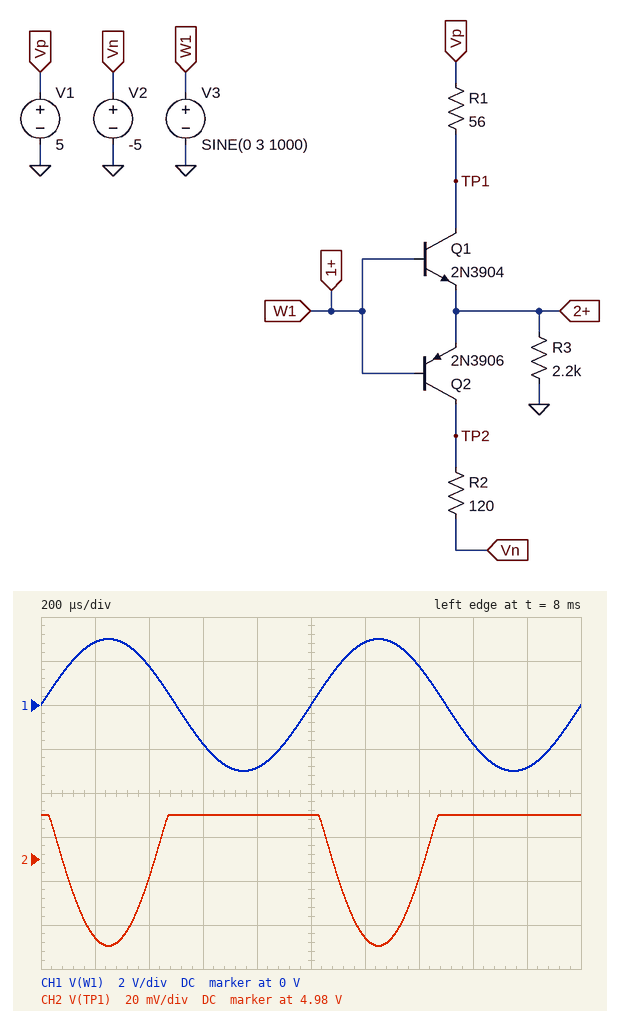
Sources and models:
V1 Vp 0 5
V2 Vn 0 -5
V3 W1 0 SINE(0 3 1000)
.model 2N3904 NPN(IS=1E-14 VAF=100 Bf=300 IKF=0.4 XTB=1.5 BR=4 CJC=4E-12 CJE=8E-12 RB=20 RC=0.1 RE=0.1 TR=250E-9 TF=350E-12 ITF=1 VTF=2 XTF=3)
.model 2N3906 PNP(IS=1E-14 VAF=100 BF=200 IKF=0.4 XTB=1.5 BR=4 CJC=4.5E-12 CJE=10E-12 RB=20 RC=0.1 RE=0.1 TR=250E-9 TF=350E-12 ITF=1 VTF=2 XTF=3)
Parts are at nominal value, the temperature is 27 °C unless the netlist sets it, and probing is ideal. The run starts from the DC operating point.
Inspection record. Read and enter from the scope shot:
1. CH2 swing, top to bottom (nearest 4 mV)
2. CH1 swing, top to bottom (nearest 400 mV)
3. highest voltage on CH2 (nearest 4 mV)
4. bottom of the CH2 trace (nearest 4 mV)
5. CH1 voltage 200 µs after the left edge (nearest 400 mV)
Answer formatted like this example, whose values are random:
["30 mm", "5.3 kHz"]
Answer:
["60 mV", "6.0 V", "5.000 V", "4.940 V", "2.8 V"]
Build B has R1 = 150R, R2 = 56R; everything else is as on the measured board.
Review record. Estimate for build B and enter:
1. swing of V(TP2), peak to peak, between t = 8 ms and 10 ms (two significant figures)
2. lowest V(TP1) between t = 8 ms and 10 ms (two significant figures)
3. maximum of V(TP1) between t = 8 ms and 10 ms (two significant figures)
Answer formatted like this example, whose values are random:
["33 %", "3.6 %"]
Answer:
["59 mV", "4.8 V", "5.0 V"]
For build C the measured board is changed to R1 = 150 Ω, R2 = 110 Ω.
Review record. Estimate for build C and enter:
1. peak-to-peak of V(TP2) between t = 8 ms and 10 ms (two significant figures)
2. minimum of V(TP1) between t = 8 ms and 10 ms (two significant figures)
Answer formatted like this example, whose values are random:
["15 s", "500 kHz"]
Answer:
["120 mV", "4.8 V"]
